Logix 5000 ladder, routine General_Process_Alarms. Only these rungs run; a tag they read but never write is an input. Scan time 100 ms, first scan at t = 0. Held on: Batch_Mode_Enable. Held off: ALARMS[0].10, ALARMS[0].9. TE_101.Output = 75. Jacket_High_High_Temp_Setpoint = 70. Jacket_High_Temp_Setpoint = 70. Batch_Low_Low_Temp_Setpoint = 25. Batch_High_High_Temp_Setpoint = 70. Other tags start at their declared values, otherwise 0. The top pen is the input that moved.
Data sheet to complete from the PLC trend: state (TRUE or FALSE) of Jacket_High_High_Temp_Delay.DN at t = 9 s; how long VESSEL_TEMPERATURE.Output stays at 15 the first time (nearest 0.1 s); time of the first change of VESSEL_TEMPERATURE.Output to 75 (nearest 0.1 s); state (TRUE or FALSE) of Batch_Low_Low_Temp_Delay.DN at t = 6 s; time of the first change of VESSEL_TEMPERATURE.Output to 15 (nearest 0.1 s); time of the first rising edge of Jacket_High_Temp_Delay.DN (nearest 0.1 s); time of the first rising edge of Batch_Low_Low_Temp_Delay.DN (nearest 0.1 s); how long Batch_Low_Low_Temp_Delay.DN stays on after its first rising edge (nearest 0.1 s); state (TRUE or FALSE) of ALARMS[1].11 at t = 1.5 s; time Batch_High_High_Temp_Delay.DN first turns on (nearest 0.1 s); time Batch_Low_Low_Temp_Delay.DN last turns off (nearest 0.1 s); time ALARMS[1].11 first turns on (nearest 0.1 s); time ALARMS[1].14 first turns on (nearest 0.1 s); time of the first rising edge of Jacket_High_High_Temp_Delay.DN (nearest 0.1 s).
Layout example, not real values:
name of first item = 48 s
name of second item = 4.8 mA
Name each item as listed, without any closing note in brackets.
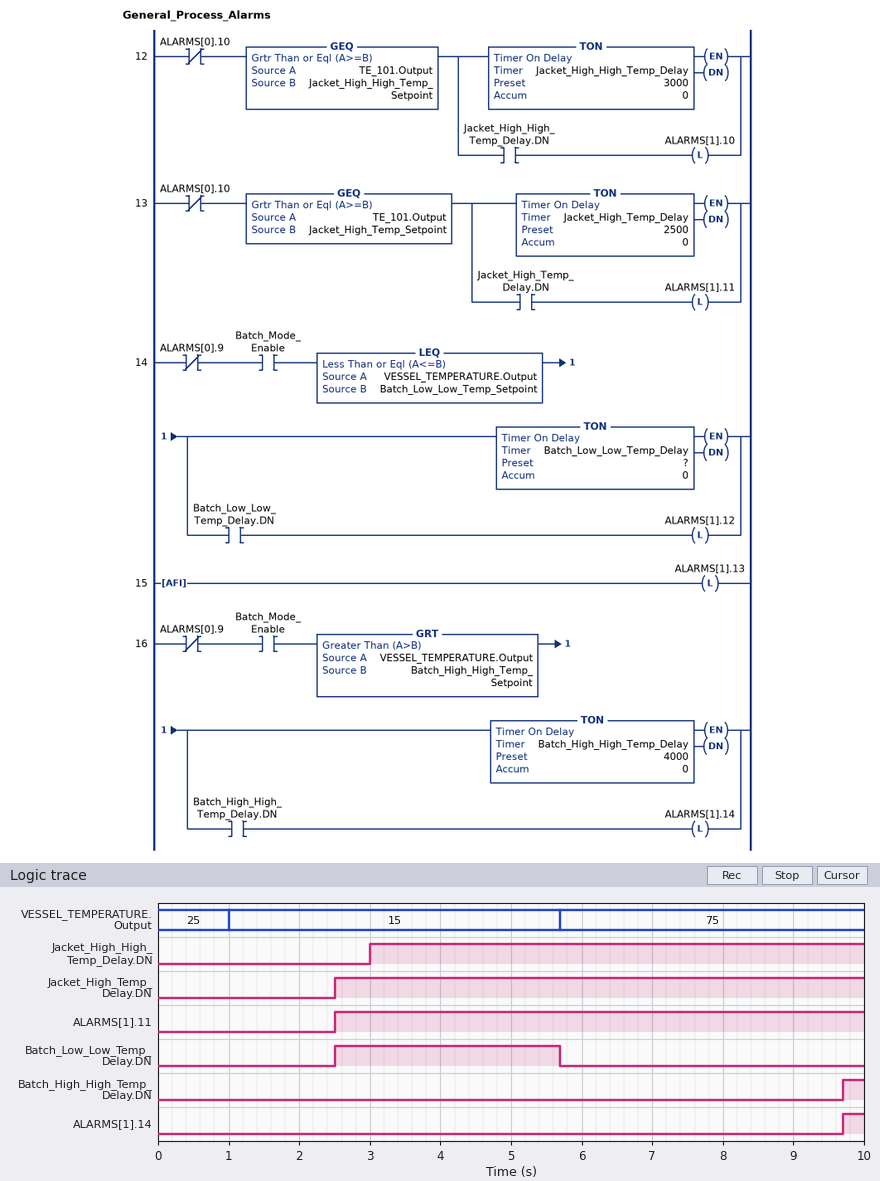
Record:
state (TRUE or FALSE) of Jacket_High_High_Temp_Delay.DN at t = 9 s = TRUE
how long VESSEL_TEMPERATURE.Output stays at 15 the first time = 4.7 s
time of the first change of VESSEL_TEMPERATURE.Output to 75 = 5.7 s
state (TRUE or FALSE) of Batch_Low_Low_Temp_Delay.DN at t = 6 s = FALSE
time of the first change of VESSEL_TEMPERATURE.Output to 15 = 1.0 s
time of the first rising edge of Jacket_High_Temp_Delay.DN = 2.5 s
time of the first rising edge of Batch_Low_Low_Temp_Delay.DN = 2.5 s
how long Batch_Low_Low_Temp_Delay.DN stays on after its first rising edge = 3.2 s
state (TRUE or FALSE) of ALARMS[1].11 at t = 1.5 s = FALSE
time Batch_High_High_Temp_Delay.DN first turns on = 9.7 s
time Batch_Low_Low_Temp_Delay.DN last turns off = 5.7 s
time ALARMS[1].11 first turns on = 2.5 s
time ALARMS[1].14 first turns on = 9.7 s
time of the first rising edge of Jacket_High_High_Temp_Delay.DN = 3.0 s
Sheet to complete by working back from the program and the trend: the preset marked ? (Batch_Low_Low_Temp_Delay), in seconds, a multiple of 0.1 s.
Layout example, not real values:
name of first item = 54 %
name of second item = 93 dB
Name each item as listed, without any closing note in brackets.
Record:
the preset marked ? (Batch_Low_Low_Temp_Delay), in seconds, a multiple of 0.1 s = 2.5 s
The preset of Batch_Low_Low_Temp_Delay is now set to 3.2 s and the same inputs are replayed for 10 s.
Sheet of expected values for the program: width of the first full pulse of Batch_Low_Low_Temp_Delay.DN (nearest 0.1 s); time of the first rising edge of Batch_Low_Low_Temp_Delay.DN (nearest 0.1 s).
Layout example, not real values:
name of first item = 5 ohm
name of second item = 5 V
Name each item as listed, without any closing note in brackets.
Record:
width of the first full pulse of Batch_Low_Low_Temp_Delay.DN = 2.5 s
time of the first rising edge of Batch_Low_Low_Temp_Delay.DN = 3.2 s
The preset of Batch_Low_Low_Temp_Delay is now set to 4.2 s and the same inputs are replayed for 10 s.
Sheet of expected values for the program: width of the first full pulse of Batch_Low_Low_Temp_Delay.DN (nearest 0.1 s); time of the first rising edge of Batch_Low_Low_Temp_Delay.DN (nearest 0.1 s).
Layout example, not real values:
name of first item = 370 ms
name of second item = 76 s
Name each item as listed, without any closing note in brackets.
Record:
width of the first full pulse of Batch_Low_Low_Temp_Delay.DN = 1.5 s
time of the first rising edge of Batch_Low_Low_Temp_Delay.DN = 4.2 s
